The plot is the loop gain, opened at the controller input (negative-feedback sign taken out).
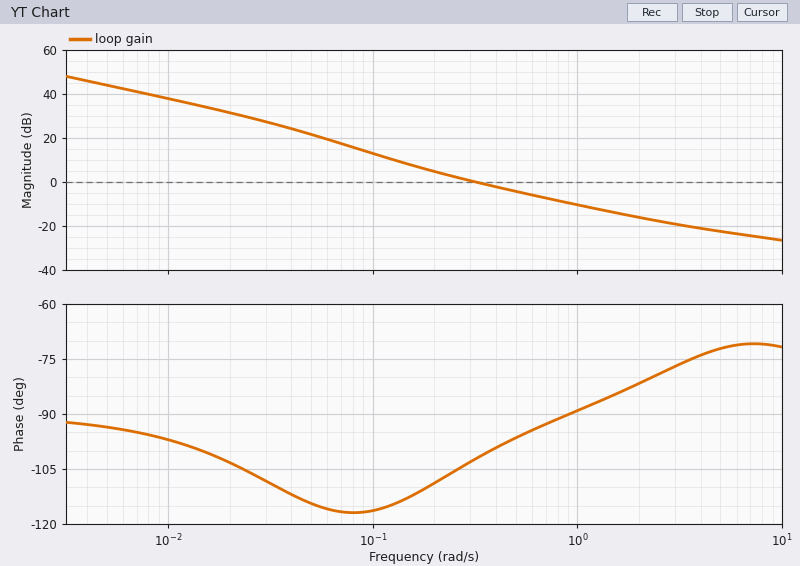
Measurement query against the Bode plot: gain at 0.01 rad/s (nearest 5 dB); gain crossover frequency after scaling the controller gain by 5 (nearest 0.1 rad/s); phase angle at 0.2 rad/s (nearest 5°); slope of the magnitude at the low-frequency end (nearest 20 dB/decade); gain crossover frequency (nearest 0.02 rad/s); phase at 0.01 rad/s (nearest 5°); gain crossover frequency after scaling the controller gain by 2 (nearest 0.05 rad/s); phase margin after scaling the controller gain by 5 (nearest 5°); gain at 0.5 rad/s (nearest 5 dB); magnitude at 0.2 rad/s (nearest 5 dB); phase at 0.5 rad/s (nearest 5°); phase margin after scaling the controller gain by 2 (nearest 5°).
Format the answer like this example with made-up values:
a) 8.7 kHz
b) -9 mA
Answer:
a) 40 dB
b) 1.5 rad/s
c) -110°
d) -20 dB/decade
e) 0.32 rad/s
f) -95°
g) 0.60 rad/s
h) 95°
i) -5 dB
j) 5 dB
k) -95°
l) 85°
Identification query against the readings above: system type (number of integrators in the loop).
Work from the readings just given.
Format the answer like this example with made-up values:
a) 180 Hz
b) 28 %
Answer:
a) 1
